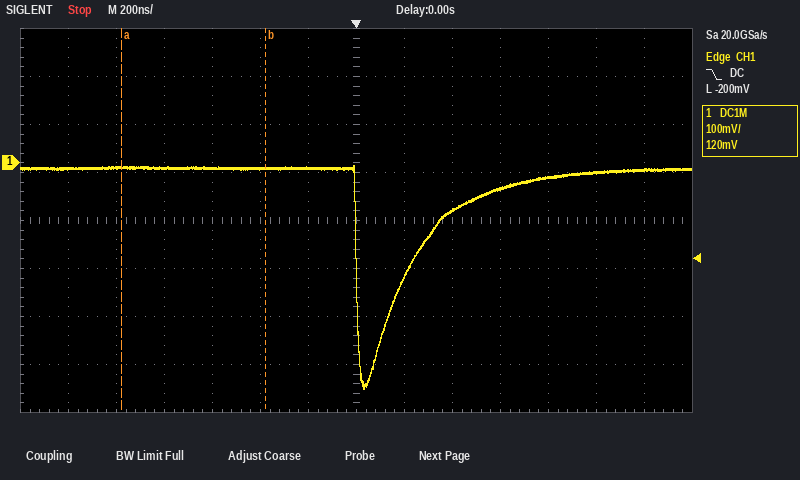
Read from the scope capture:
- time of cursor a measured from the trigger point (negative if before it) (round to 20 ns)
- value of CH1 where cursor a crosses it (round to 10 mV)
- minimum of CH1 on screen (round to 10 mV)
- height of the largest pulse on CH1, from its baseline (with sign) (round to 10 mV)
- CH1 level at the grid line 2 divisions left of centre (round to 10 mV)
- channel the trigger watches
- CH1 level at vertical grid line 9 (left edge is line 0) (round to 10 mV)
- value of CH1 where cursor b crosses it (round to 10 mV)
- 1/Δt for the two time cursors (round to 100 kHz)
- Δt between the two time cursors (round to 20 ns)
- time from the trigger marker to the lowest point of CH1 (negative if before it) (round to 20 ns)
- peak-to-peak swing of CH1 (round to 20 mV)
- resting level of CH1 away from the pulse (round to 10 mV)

-980 ns
-10 mV
-470 mV
-460 mV
-10 mV
CH1
-100 mV
-10 mV
1.7 MHz
600 ns
+40 ns
460 mV
-10 mV
